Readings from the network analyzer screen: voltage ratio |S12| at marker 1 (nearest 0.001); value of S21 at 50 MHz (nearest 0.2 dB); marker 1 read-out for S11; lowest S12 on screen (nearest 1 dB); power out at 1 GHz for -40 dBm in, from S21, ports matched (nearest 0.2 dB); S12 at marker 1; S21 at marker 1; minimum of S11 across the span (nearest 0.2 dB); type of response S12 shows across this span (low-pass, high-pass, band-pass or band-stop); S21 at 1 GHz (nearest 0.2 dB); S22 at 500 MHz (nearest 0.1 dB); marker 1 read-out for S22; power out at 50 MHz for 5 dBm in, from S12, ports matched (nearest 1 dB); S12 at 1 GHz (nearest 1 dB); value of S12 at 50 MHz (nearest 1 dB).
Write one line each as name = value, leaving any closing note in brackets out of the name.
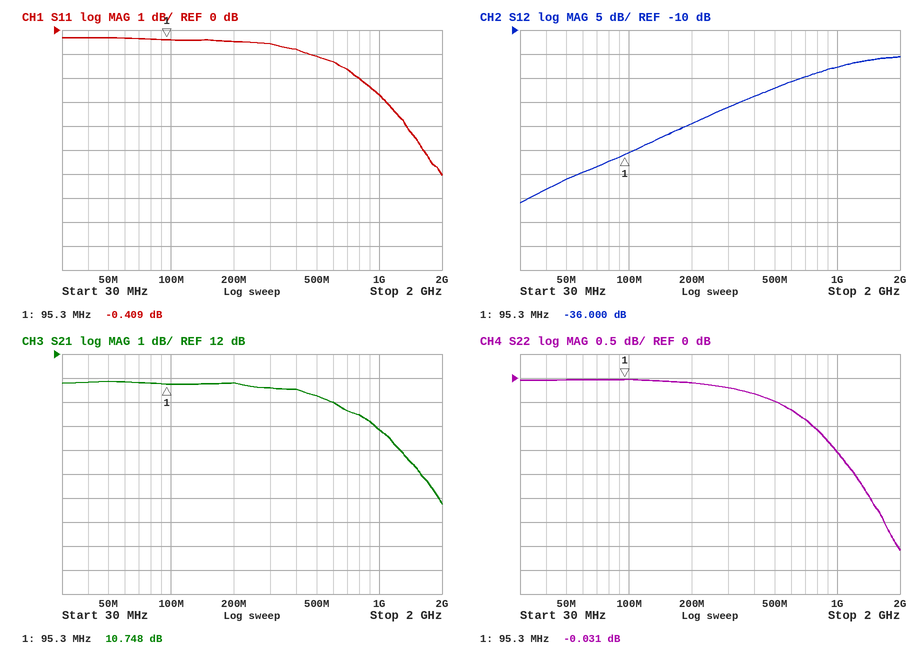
voltage ratio |S12| at marker 1 = 0.016
value of S21 at 50 MHz = 10.8 dB
marker 1 read-out for S11 = -0.409 dB
lowest S12 on screen = -46 dB
power out at 1 GHz for -40 dBm in, from S21, ports matched = -31.2 dBm
S12 at marker 1 = -36.000 dB
S21 at marker 1 = 10.748 dB
minimum of S11 across the span = -6.0 dB
type of response S12 shows across this span = high-pass
S21 at 1 GHz = 8.8 dB
S22 at 500 MHz = -0.5 dB
marker 1 read-out for S22 = -0.031 dB
power out at 50 MHz for 5 dBm in, from S12, ports matched = -36 dBm
S12 at 1 GHz = -18 dB
value of S12 at 50 MHz = -41 dB
